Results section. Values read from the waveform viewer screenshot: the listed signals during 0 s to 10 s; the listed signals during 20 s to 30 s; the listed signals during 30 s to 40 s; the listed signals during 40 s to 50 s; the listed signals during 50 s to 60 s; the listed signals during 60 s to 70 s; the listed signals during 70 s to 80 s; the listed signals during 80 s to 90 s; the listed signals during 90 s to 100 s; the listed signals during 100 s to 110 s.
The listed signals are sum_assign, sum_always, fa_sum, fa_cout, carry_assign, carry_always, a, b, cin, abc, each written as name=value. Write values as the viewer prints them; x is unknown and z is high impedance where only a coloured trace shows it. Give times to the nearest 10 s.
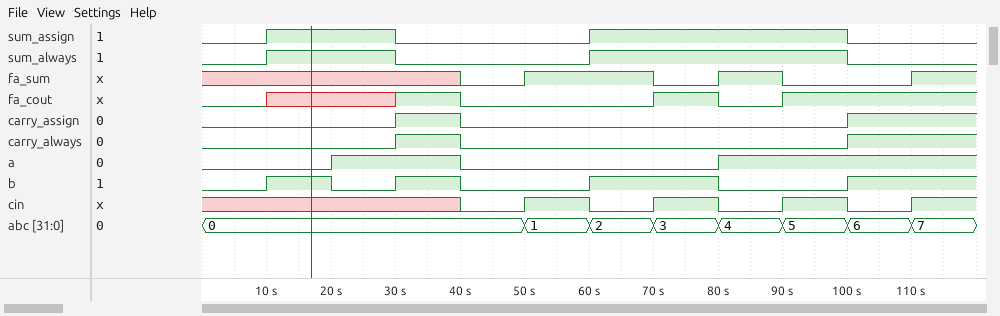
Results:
sum_assign=0, sum_always=0, fa_sum=x, fa_cout=0, carry_assign=0, carry_always=0, a=0, b=0, cin=x, abc=0
sum_assign=1, sum_always=1, fa_sum=x, fa_cout=x, carry_assign=0, carry_always=0, a=1, b=0, cin=x, abc=0
sum_assign=0, sum_always=0, fa_sum=x, fa_cout=1, carry_assign=1, carry_always=1, a=1, b=1, cin=x, abc=0
sum_assign=0, sum_always=0, fa_sum=0, fa_cout=0, carry_assign=0, carry_always=0, a=0, b=0, cin=0, abc=0
sum_assign=0, sum_always=0, fa_sum=1, fa_cout=0, carry_assign=0, carry_always=0, a=0, b=0, cin=1, abc=1
sum_assign=1, sum_always=1, fa_sum=1, fa_cout=0, carry_assign=0, carry_always=0, a=0, b=1, cin=0, abc=2
sum_assign=1, sum_always=1, fa_sum=0, fa_cout=1, carry_assign=0, carry_always=0, a=0, b=1, cin=1, abc=3
sum_assign=1, sum_always=1, fa_sum=1, fa_cout=0, carry_assign=0, carry_always=0, a=1, b=0, cin=0, abc=4
sum_assign=1, sum_always=1, fa_sum=0, fa_cout=1, carry_assign=0, carry_always=0, a=1, b=0, cin=1, abc=5
sum_assign=0, sum_always=0, fa_sum=0, fa_cout=1, carry_assign=1, carry_always=1, a=1, b=1, cin=0, abc=6
